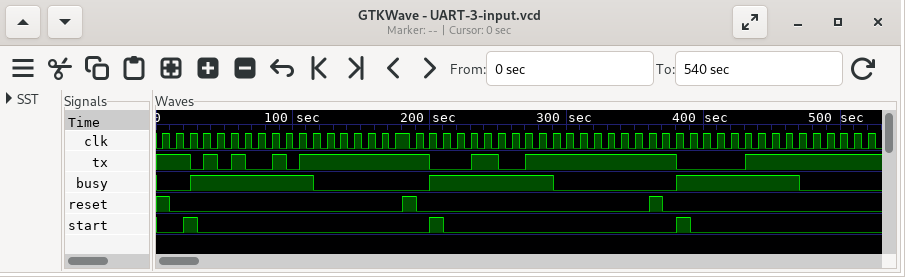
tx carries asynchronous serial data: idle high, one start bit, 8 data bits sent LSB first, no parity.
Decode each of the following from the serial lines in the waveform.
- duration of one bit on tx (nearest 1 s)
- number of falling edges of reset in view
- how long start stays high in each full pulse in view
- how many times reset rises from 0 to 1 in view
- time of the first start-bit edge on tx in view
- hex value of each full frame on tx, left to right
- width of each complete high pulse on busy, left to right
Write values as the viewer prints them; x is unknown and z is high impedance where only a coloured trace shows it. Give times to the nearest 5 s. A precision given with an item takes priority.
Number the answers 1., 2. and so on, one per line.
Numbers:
1. 10 s
2. 3
3. 10 s, 10 s, 10 s
4. 2
5. 25 s
6. A5, CC, F0
7. 90 s, 90 s, 90 s
